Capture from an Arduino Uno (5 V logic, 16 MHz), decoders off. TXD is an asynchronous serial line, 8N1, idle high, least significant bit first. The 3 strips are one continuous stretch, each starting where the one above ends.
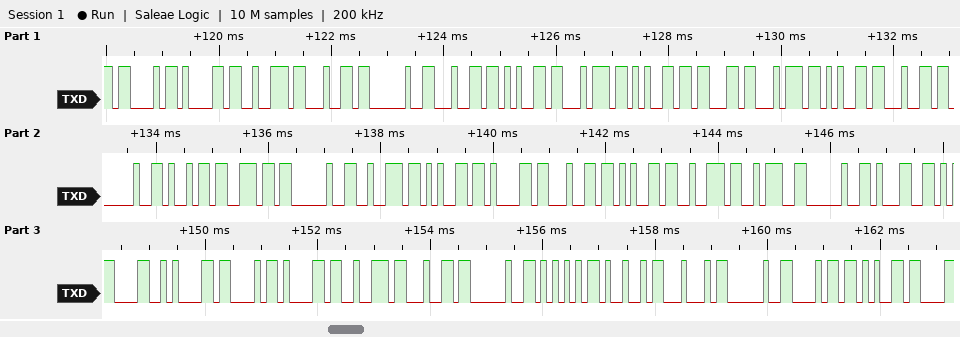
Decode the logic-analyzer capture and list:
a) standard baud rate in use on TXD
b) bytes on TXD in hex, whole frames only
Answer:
9600 baud
0x43 0x61 0x72 0x64 0x20 0x64 0x65 0x74 0x65 0x63 0x74 0x65 0x64 0x20 0x69 0x6E 0x20 0x72 0x65 0x61 0x64 0x65 0x72 0x3A 0x20 0x31 0x0D 0x0A 0x43 0x61 0x72 0x64 0x20 0x55 0x49 0x44 0x20 0x68 0x65
